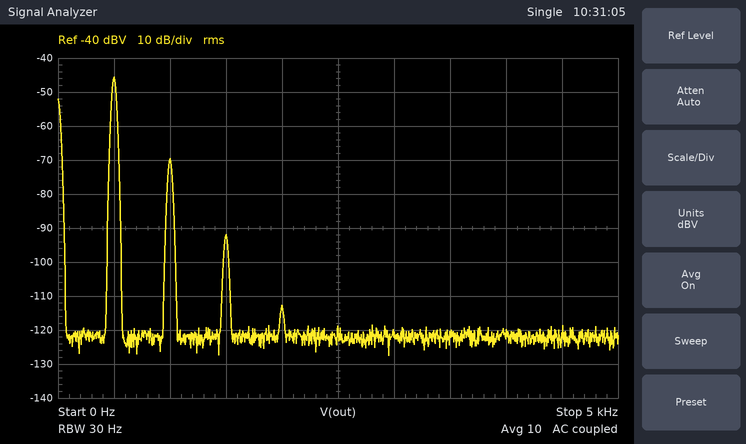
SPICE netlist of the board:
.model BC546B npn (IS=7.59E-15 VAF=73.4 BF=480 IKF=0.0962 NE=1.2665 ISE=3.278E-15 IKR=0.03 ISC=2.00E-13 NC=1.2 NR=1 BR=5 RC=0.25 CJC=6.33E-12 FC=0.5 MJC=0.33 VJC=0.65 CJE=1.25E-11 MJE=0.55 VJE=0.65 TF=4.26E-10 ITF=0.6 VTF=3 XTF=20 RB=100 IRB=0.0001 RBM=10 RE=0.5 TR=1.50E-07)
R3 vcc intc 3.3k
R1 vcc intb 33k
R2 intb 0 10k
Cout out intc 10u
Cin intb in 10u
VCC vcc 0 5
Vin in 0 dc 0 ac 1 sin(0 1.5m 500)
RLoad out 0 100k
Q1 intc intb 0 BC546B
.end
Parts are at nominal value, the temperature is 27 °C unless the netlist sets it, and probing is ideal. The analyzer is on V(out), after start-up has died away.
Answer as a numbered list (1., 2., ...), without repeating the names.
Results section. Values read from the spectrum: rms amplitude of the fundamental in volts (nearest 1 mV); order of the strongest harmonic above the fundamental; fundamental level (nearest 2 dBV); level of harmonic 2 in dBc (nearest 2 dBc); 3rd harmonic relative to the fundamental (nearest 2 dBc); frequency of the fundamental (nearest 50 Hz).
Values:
1. 5 mV
2. 2
3. -46 dBV
4. -24 dBc
5. -46 dBc
6. 500 Hz
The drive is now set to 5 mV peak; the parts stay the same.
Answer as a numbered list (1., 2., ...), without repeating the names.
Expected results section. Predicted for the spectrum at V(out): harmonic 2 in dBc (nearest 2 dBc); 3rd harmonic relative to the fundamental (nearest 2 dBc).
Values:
1. -12 dBc
2. -22 dBc
